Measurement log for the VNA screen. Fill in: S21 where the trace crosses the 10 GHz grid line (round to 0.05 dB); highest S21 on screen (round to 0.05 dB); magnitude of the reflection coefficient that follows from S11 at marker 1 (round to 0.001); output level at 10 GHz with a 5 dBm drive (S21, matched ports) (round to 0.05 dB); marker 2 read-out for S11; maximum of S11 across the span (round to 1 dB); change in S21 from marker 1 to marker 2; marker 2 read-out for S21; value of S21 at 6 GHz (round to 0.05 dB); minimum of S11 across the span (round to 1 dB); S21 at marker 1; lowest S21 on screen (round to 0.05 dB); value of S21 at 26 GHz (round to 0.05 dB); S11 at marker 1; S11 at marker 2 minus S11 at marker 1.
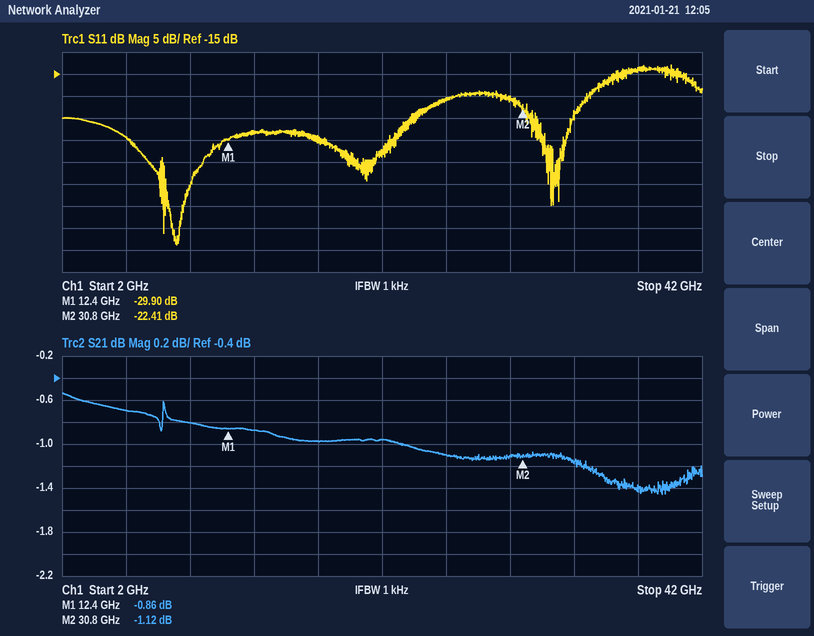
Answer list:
-0.80 dB
-0.55 dB
0.032
4.20 dBm
-22.41 dB
-13 dB
-0.26 dB
-1.12 dB
-0.70 dB
-54 dB
-0.86 dB
-1.45 dB
-1.10 dB
-29.90 dB
7.49 dB
